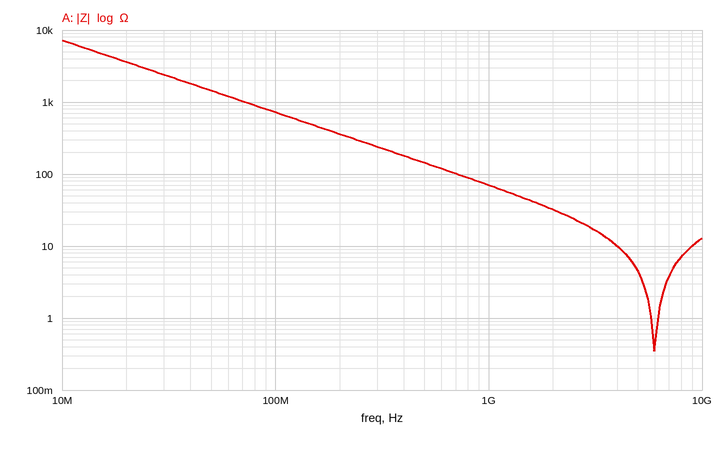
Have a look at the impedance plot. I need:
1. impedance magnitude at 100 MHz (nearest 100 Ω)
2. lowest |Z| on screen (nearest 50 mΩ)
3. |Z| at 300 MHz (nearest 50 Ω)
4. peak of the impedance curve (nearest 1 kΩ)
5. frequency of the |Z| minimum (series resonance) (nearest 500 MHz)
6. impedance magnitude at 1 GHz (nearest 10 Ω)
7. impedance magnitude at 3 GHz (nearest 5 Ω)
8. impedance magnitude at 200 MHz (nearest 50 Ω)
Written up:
700 Ω
350 mΩ
250 Ω
7 kΩ
6.0 GHz
70 Ω
20 Ω
350 Ω
